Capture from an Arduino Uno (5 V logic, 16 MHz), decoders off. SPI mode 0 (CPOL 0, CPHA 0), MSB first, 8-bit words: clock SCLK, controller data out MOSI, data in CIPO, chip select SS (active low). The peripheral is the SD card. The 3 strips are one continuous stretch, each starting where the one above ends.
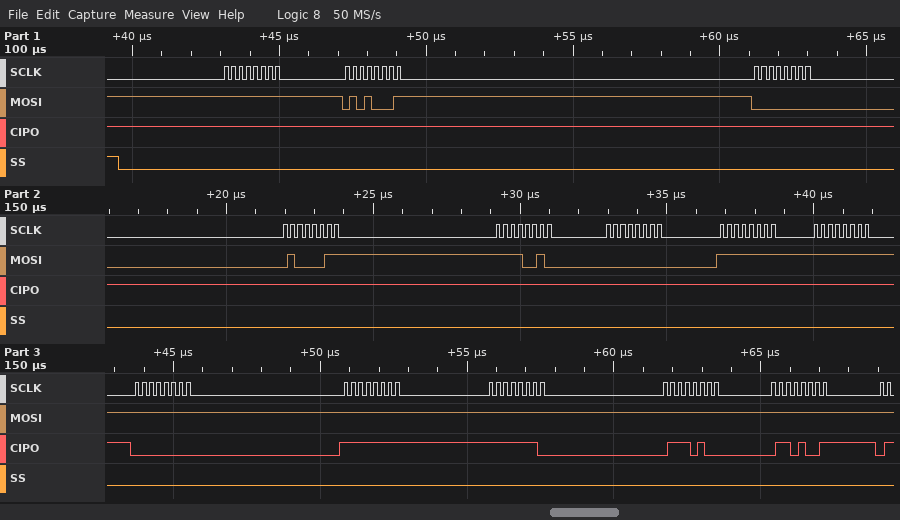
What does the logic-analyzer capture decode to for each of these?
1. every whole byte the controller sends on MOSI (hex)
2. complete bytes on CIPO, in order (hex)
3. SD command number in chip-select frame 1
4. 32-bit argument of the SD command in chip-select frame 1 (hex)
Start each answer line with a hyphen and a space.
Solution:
- FF 51 00 43 F2 00 FF FF FF FF FF FF FF
- FF FF FF FF FF FF FF FF 00 FF FE 74 69
- CMD17
- 0x0043F200
